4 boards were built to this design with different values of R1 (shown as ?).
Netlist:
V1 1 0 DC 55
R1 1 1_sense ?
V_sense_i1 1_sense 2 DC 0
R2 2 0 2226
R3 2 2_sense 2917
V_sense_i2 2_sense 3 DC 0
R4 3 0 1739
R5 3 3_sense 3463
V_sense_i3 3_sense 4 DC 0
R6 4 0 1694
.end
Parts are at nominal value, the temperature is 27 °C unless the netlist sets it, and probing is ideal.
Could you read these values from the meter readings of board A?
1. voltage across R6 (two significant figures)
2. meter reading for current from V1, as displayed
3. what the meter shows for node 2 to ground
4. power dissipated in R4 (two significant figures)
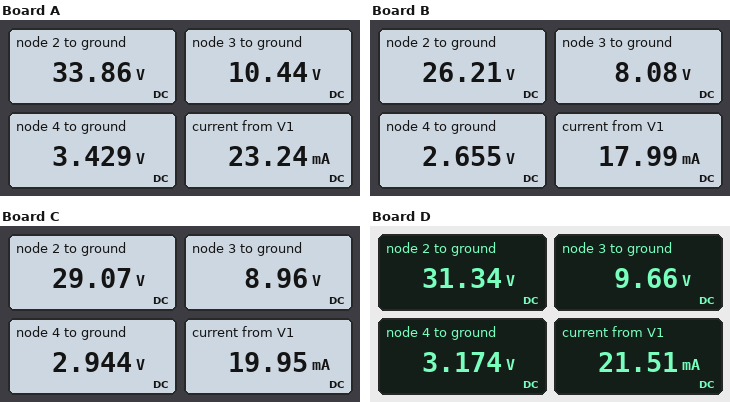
3.4 V
23.24 mA
33.86 V
63 mW
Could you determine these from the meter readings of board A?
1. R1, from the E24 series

910 Ω
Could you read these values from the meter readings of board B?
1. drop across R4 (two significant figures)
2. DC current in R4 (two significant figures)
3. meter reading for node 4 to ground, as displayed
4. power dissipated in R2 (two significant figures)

8.1 V
4.6 mA
2.655 V
310 mW
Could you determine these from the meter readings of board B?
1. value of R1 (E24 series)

1.6 kΩ
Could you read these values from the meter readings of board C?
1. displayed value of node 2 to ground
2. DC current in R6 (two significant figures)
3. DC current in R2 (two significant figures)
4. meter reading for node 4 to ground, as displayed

29.07 V
1.7 mA
13 mA
2.944 V
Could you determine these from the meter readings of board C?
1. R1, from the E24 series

1.3 kΩ
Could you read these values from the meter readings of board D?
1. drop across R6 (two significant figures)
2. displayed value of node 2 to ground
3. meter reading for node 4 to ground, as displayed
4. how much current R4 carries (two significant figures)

3.2 V
31.34 V
3.174 V
5.6 mA
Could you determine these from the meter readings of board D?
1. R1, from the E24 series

1.1 kΩ
